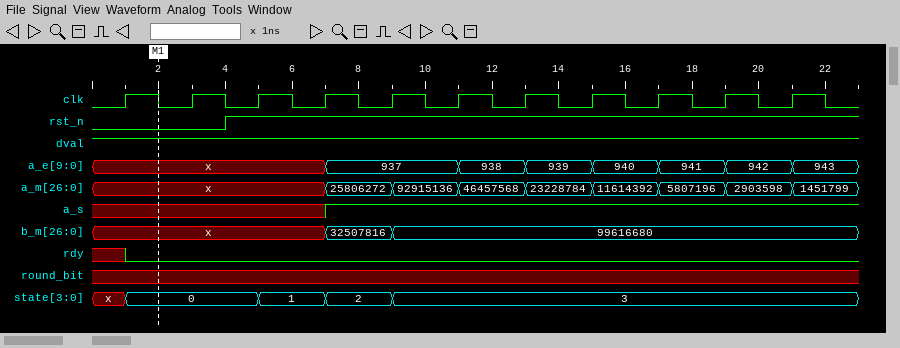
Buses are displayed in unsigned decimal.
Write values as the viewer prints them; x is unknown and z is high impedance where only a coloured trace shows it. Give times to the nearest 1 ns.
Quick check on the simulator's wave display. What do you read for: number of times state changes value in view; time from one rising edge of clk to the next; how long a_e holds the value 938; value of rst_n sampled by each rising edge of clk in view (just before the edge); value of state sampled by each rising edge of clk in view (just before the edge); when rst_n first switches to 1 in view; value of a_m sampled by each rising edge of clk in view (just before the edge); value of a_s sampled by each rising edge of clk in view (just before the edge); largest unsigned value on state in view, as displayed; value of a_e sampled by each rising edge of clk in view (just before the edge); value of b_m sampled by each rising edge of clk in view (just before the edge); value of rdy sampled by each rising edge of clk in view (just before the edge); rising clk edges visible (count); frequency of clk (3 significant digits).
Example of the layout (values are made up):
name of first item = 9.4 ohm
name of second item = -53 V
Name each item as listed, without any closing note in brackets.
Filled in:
number of times state changes value in view = 4
time from one rising edge of clk to the next = 2 ns
how long a_e holds the value 938 = 2 ns
value of rst_n sampled by each rising edge of clk in view = 0 0 1 1 1 1 1 1 1 1 1
value of state sampled by each rising edge of clk in view = x, 0, 0, 1, 2, 3, 3, 3, 3, 3, 3
when rst_n first switches to 1 in view = 4 ns
value of a_m sampled by each rising edge of clk in view = x, x, x, x, 25806272, 92915136, 46457568, 23228784, 11614392, 5807196, 2903598
value of a_s sampled by each rising edge of clk in view = x x x x 1 1 1 1 1 1 1
largest unsigned value on state in view, as displayed = 3
value of a_e sampled by each rising edge of clk in view = x, x, x, x, 937, 937, 938, 939, 940, 941, 942
value of b_m sampled by each rising edge of clk in view = x, x, x, x, 32507816, 99616680, 99616680, 99616680, 99616680, 99616680, 99616680
value of rdy sampled by each rising edge of clk in view = x 0 0 0 0 0 0 0 0 0 0
rising clk edges visible = 11
frequency of clk = 500 MHz
